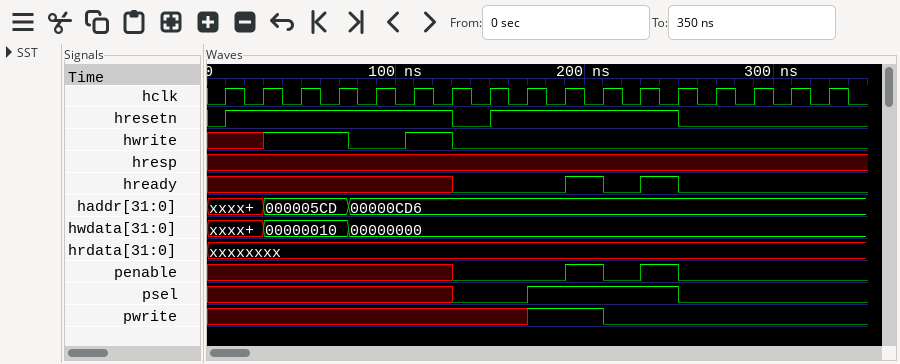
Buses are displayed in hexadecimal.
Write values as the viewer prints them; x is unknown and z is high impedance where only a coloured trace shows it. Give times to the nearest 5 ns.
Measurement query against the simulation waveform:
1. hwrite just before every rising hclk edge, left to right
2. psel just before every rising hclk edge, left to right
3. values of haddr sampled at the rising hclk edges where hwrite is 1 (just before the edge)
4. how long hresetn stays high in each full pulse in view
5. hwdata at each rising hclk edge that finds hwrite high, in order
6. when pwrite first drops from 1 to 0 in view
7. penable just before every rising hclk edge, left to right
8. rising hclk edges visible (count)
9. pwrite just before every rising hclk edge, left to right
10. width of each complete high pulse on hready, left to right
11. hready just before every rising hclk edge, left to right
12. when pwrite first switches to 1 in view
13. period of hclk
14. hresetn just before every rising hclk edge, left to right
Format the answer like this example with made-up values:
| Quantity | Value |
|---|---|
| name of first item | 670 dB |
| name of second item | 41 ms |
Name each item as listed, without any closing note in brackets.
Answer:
| Quantity | Value |
|---|---|
| hwrite just before every rising hclk edge, left to right | x x 1 1 0 1 1 0 0 0 0 0 0 0 0 0 0 |
| psel just before every rising hclk edge, left to right | x x x x x x x 0 0 1 1 1 1 0 0 0 0 |
| values of haddr sampled at the rising hclk edges where hwrite is 1 | 000005CD, 000005CD, 00000CD6, 00000CD6 |
| how long hresetn stays high in each full pulse in view | 120 ns, 100 ns |
| hwdata at each rising hclk edge that finds hwrite high, in order | 00000010, 00000010, 00000000, 00000000 |
| when pwrite first drops from 1 to 0 in view | 210 ns |
| penable just before every rising hclk edge, left to right | x x x x x x x 0 0 0 1 0 1 0 0 0 0 |
| rising hclk edges visible | 17 |
| pwrite just before every rising hclk edge, left to right | x x x x x x x x x 1 1 0 0 0 0 0 0 |
| width of each complete high pulse on hready, left to right | 20 ns, 20 ns |
| hready just before every rising hclk edge, left to right | x x x x x x x 0 0 0 1 0 1 0 0 0 0 |
| when pwrite first switches to 1 in view | 170 ns |
| period of hclk | 20 ns |
| hresetn just before every rising hclk edge, left to right | 0 1 1 1 1 1 1 0 1 1 1 1 1 0 0 0 0 |
